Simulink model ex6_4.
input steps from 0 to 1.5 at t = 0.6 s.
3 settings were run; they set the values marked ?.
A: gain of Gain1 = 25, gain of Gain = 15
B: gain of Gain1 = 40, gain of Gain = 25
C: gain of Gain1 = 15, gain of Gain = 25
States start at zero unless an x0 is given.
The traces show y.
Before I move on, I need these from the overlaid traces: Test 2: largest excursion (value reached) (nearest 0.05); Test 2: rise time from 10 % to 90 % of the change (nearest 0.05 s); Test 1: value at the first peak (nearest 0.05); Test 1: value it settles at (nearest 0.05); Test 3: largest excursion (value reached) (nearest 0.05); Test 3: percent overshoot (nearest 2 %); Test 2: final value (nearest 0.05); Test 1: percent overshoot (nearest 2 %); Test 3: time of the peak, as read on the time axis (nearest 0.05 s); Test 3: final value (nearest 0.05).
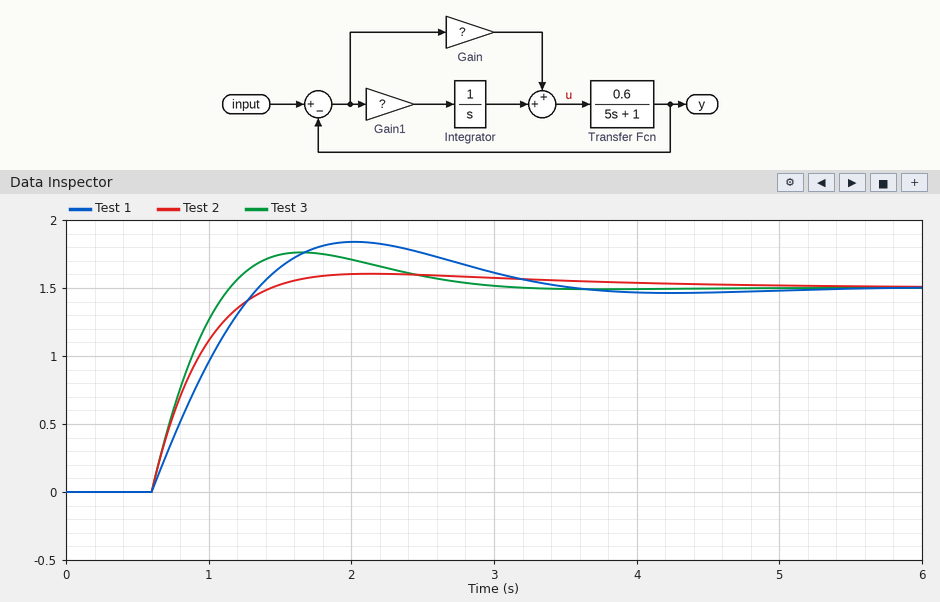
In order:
1.60
0.55 s
1.85
1.50
1.75
18 %
1.50
22 %
1.65 s
1.50
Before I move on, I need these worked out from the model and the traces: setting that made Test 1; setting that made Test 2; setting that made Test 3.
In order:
A
C
B
